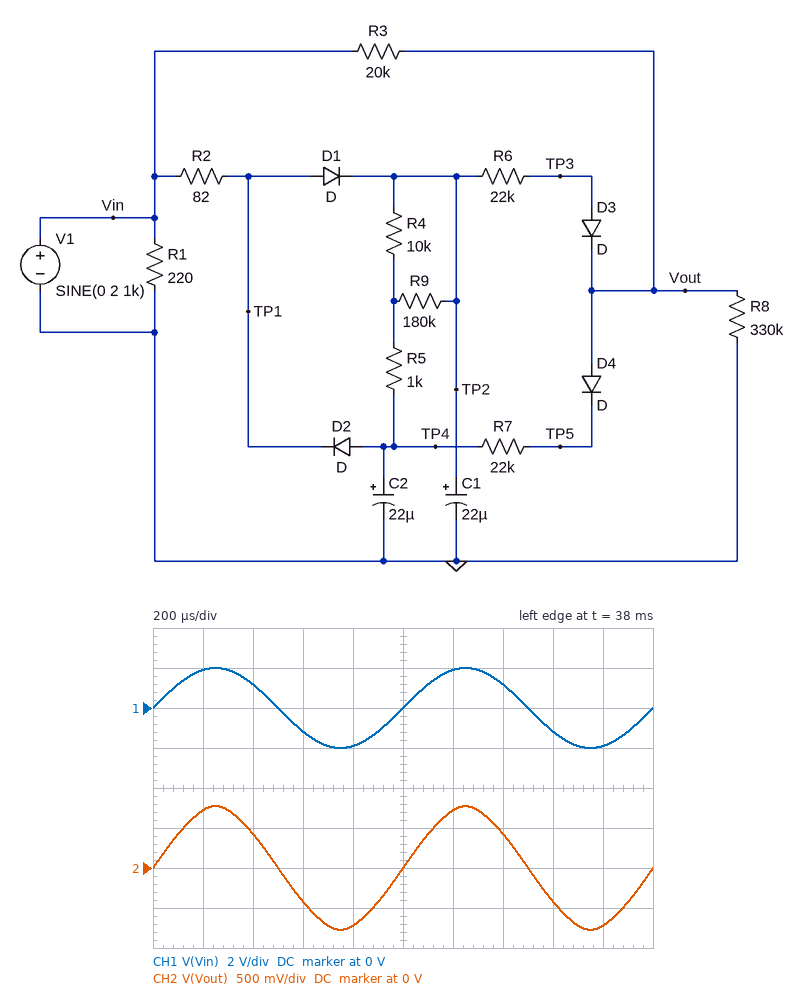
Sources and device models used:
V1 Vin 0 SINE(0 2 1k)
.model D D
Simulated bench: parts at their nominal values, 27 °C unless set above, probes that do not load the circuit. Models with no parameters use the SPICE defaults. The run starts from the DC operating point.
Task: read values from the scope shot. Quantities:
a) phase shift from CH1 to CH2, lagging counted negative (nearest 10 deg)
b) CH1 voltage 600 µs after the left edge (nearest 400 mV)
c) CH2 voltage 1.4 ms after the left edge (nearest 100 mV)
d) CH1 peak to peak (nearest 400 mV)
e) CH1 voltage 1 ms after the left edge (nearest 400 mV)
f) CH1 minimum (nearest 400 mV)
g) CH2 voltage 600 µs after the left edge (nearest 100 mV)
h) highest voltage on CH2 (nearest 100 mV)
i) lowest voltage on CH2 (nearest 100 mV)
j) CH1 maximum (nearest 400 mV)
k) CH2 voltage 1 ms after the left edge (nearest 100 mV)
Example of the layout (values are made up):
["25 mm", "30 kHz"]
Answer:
["0 deg", "-1.2 V", "400 mV", "4.0 V", "0 V", "-2.0 V", "-400 mV", "800 mV", "-800 mV", "2.0 V", "0 V"]
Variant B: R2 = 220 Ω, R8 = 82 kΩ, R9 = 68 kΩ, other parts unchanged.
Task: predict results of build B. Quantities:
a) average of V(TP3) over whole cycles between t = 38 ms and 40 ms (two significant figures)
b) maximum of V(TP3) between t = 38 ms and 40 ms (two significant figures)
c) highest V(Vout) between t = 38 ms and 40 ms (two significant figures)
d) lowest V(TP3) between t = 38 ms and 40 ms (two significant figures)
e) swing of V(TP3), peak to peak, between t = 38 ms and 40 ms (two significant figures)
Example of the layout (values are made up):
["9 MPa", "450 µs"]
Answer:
["450 mV", "880 mV", "810 mV", "-230 mV", "1.1 V"]
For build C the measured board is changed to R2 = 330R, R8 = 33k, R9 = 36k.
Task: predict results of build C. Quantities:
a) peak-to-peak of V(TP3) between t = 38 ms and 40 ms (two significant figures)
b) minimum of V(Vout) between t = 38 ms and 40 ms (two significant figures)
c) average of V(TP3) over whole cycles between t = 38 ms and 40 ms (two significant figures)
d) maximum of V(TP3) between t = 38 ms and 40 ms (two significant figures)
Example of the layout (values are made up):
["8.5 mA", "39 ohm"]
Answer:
["910 mV", "-740 mV", "410 mV", "740 mV"]
